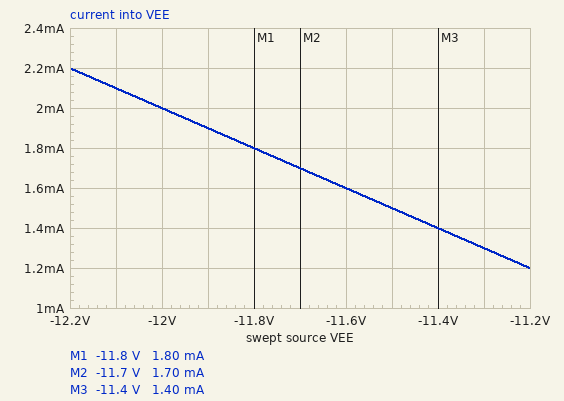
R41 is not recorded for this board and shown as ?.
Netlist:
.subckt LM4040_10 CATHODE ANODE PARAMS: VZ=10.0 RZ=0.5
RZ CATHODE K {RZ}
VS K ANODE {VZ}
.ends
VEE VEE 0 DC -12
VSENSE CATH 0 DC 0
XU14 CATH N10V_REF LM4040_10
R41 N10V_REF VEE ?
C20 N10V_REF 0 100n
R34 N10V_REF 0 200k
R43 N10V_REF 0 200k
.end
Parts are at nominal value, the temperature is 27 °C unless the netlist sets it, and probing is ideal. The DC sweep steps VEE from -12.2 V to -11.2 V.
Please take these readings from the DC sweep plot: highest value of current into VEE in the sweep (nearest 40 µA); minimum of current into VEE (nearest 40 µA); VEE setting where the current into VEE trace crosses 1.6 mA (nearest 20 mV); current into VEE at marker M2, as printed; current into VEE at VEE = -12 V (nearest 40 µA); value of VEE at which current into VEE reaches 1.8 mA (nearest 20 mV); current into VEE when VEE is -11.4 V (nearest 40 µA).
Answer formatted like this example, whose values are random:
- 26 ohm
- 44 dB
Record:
- 2.20 mA
- 1.20 mA
- -11.60 V
- 1.70 mA
- 2.00 mA
- -11.80 V
- 1.40 mA
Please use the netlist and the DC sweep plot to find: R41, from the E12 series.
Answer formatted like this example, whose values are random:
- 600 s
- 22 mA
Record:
- 1 kΩ
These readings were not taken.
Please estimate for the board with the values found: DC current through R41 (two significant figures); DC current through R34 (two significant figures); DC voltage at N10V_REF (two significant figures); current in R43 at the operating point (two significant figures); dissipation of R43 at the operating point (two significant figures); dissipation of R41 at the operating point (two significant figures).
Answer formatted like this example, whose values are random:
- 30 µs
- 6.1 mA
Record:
- 2.0 mA
- 50 µA
- -10 V
- 50 µA
- 500 µW
- 4.0 mW
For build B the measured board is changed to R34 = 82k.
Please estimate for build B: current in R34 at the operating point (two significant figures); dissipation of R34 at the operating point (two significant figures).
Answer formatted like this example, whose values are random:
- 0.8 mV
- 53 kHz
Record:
- 120 µA
- 1.2 mW
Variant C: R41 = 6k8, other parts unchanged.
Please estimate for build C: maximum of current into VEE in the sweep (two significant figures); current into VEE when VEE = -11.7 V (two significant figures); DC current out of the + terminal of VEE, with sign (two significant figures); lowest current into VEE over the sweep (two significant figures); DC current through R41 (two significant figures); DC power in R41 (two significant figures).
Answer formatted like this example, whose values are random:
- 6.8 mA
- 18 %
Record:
- 320 µA
- 250 µA
- -290 µA
- 180 µA
- 290 µA
- 590 µW
